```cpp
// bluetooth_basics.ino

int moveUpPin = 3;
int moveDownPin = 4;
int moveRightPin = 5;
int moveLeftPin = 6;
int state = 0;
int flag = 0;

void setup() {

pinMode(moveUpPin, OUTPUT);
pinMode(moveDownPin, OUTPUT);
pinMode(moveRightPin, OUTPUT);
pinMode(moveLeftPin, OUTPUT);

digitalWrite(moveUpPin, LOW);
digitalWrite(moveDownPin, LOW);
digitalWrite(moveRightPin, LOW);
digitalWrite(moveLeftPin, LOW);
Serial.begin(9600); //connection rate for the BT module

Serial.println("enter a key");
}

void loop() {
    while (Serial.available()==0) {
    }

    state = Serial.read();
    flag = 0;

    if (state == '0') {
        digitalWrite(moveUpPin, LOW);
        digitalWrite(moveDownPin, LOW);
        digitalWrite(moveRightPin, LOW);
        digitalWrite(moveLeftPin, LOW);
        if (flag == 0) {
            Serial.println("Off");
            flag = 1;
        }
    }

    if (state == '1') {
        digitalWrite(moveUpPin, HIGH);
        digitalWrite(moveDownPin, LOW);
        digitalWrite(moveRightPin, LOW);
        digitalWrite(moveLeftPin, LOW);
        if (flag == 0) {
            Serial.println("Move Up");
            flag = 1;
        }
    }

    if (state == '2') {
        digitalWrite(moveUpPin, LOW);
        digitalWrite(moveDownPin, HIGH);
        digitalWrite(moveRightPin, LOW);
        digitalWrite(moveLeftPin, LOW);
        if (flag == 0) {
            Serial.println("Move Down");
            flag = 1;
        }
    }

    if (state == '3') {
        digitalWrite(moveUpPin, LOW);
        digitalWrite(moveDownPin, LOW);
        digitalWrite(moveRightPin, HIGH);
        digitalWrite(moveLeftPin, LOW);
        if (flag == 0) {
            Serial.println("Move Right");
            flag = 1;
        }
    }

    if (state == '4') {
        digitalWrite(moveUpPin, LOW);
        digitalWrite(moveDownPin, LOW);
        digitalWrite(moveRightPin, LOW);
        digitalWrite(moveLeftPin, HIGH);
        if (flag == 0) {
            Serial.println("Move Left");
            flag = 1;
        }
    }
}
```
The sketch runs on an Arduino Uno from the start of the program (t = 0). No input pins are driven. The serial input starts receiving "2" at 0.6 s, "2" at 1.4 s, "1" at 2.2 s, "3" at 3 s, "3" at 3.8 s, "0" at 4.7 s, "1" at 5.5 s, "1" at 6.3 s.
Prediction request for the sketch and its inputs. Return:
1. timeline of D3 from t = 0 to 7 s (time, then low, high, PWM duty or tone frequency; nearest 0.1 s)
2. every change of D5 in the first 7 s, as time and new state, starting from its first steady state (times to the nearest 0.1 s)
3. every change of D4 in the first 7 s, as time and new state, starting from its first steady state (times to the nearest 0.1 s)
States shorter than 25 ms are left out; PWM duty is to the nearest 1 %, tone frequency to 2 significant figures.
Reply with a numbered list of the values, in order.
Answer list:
1. 0 s low; 2.2 s high; 3 s low; 5.5 s high
2. 0 s low; 3 s high; 4.7 s low
3. 0 s low; 0.6 s high; 2.2 s low
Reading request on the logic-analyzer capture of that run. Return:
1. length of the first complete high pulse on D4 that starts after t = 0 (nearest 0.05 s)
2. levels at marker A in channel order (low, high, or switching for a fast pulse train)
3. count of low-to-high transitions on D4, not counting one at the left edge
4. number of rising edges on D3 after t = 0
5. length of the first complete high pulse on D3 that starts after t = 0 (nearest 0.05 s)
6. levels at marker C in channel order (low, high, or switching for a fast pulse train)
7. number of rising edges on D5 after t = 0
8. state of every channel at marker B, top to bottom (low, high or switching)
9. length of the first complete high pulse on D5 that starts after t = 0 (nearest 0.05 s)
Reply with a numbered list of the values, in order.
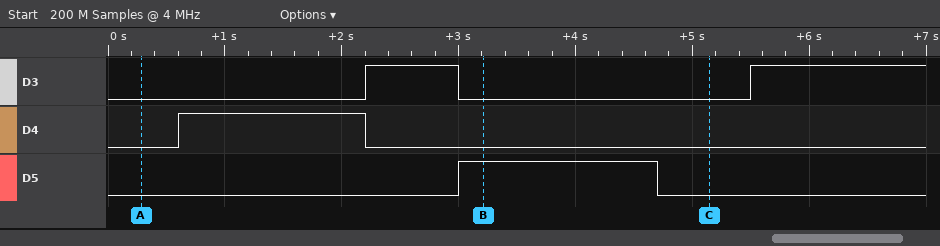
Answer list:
1. 1.60 s
2. D3 low, D4 low, D5 low
3. 1
4. 2
5. 0.80 s
6. D3 low, D4 low, D5 low
7. 1
8. D3 low, D4 low, D5 high
9. 1.70 s
